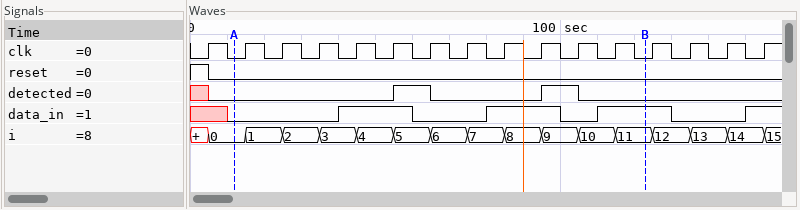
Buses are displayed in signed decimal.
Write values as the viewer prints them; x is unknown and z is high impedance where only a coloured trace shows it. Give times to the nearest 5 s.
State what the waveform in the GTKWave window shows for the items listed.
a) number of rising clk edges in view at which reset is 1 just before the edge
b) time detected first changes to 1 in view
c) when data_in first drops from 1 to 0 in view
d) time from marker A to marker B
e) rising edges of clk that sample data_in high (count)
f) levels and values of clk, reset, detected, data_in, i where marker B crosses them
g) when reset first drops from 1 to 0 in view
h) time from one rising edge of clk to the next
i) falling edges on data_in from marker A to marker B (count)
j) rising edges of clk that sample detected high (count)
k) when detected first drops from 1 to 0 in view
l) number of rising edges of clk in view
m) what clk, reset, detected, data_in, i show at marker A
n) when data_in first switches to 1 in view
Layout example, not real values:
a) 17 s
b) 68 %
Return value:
a) 1
b) 55 s
c) 60 s
d) 110 s
e) 7
f) clk=0, reset=0, detected=0, data_in=1, i=11
g) 5 s
h) 10 s
i) 2
j) 2
k) 65 s
l) 16
m) clk=0, reset=0, detected=0, data_in=0, i=0
n) 40 s
